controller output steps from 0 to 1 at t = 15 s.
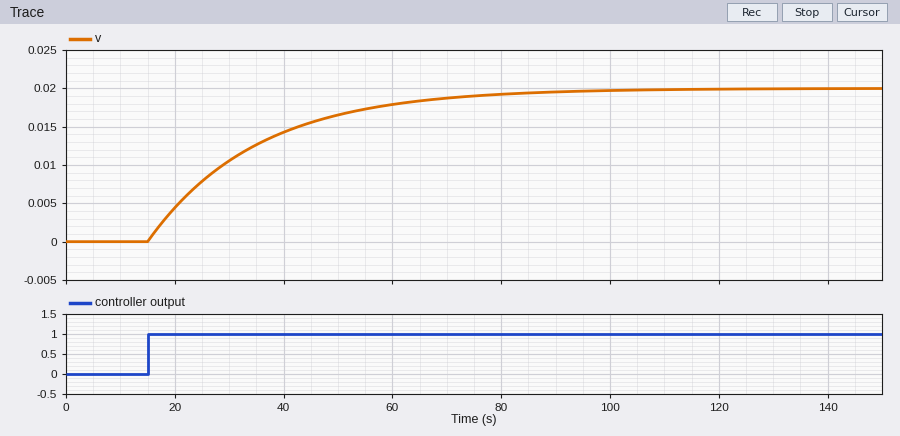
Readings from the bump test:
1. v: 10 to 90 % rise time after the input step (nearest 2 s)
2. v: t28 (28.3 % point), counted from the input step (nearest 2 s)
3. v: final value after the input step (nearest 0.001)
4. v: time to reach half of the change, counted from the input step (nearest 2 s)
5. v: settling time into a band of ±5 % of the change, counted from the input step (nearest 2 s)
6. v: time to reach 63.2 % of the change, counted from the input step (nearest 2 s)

44 s
6 s
0.020
14 s
60 s
20 s
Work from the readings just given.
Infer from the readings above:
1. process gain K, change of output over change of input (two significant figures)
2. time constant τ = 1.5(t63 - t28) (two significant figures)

0.020
21 s
